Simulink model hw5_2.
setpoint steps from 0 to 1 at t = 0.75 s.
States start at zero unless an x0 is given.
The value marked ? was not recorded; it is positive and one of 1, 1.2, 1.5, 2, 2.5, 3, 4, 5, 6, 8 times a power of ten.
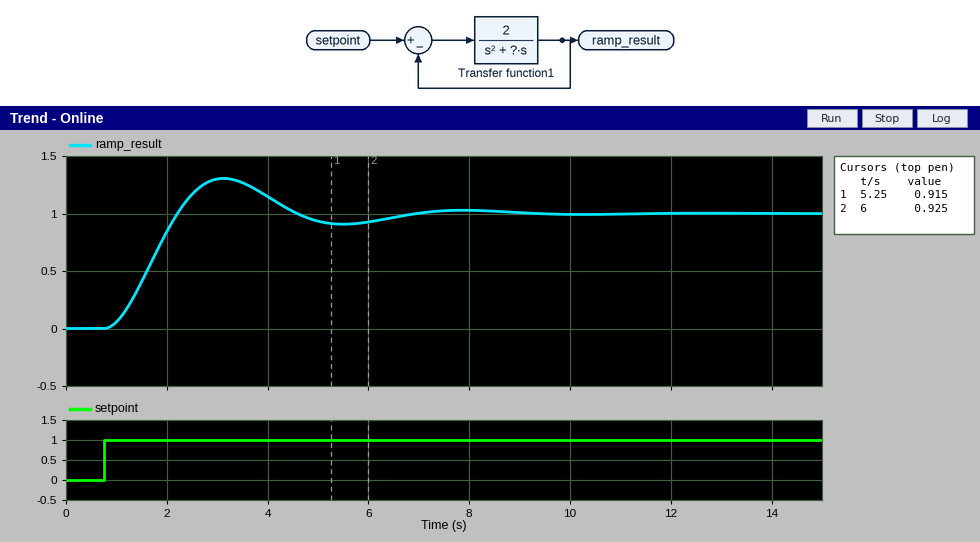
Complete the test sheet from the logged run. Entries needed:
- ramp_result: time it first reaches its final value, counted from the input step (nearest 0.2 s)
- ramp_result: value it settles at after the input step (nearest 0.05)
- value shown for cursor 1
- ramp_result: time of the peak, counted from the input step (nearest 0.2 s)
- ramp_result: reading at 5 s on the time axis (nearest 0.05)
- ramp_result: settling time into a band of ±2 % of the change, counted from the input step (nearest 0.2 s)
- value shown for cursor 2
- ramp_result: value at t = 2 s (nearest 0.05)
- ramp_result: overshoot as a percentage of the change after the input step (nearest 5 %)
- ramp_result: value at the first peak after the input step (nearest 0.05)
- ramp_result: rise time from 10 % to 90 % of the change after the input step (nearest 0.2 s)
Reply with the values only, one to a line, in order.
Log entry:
1.4 s
1.00
0.915
2.4 s
0.95
7.8 s
0.925
0.85
30 %
1.30
1.0 s
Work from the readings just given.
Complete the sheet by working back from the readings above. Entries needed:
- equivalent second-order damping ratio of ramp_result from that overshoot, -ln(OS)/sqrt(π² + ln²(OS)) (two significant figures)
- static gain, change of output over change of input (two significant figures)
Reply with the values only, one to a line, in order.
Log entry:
0.36
1.0
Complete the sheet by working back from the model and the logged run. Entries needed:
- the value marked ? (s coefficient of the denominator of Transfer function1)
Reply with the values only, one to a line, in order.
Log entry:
1
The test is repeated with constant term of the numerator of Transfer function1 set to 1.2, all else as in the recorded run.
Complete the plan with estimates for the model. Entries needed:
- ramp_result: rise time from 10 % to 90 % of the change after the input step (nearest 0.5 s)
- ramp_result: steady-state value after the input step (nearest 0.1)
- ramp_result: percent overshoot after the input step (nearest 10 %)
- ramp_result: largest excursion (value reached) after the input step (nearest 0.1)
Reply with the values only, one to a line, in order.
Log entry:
1.5 s
1.0
20 %
1.2
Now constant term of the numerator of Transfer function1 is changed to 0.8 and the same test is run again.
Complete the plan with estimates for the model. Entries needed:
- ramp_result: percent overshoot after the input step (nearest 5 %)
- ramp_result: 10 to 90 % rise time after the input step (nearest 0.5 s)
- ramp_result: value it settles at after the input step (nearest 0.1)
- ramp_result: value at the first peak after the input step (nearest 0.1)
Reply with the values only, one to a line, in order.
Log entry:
10 %
2.0 s
1.0
1.1
